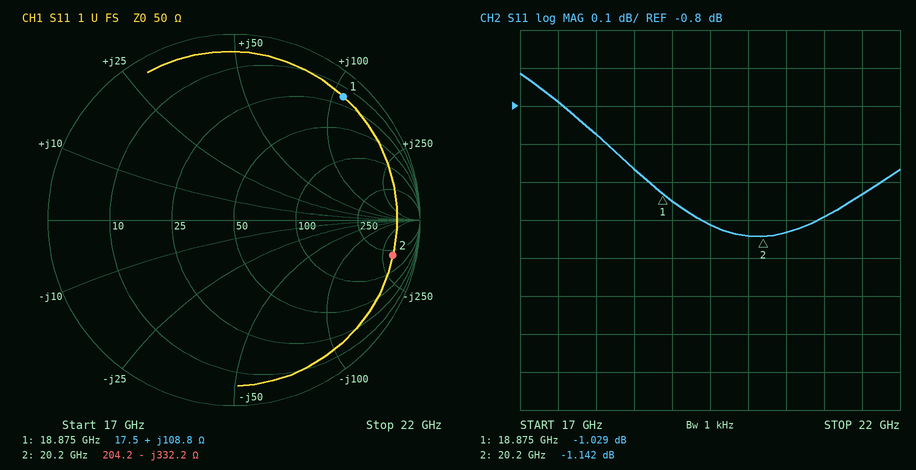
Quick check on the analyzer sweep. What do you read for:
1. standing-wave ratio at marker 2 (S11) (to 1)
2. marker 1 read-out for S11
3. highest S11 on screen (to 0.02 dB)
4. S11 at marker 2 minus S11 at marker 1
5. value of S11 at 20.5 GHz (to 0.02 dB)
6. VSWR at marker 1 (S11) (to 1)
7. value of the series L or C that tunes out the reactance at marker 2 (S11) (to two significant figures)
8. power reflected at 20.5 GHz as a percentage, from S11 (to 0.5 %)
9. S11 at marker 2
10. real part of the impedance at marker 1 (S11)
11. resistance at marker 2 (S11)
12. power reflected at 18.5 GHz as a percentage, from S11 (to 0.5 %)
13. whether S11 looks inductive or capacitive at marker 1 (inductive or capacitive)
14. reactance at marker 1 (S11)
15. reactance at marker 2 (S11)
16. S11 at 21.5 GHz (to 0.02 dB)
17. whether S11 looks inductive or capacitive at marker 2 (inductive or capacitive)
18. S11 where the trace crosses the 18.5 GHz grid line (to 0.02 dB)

15
-1.029 dB
-0.72 dB
-0.113 dB
-1.14 dB
17
2.6 nH
77.0 %
-1.142 dB
17.5 Ω
204.2 Ω
80.0 %
inductive
+108.8 Ω
-332.2 Ω
-1.04 dB
capacitive
-0.96 dB
